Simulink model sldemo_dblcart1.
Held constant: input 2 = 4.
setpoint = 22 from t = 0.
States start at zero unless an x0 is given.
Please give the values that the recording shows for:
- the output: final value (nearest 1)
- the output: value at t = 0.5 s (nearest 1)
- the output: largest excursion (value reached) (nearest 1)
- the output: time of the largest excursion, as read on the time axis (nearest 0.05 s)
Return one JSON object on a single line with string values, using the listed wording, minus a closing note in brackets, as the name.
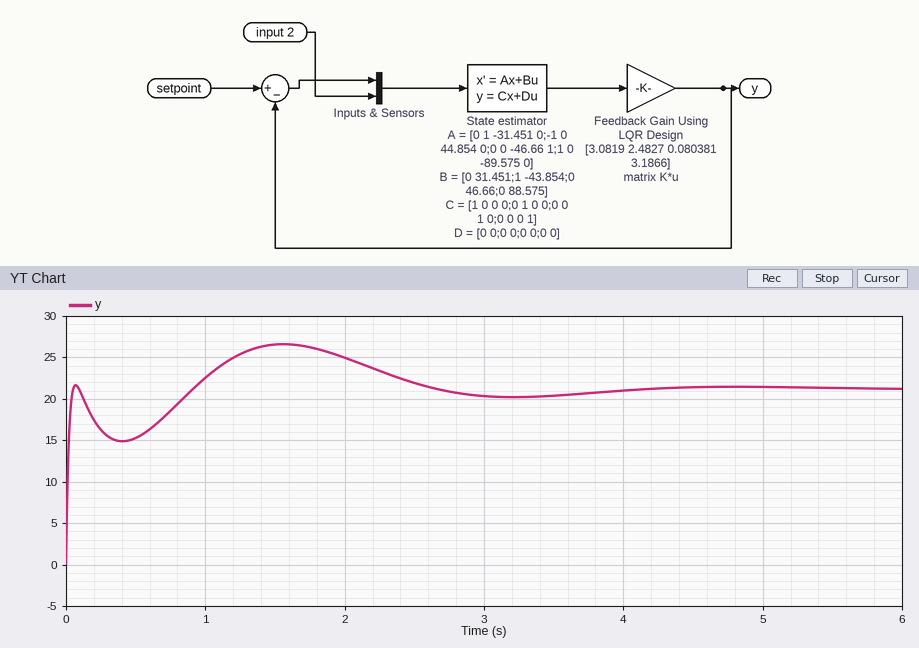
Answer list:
{"the output: final value": "21", "the output: value at t = 0.5 s": "15", "the output: largest excursion (value reached)": "27", "the output: time of the largest excursion, as read on the time axis": "1.55 s"}
